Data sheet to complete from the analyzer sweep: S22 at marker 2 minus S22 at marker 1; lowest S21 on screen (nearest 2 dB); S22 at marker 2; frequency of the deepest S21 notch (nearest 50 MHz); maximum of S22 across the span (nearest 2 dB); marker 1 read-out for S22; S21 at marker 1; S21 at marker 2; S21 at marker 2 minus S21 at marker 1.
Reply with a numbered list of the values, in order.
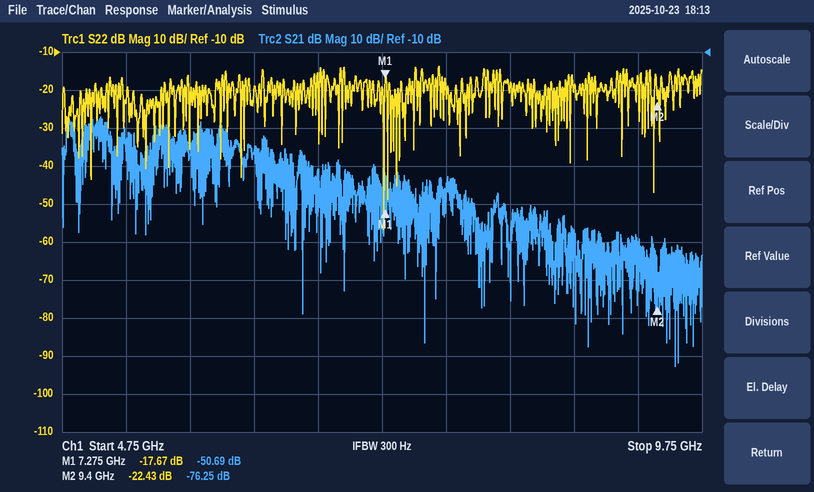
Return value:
1. -4.76 dB
2. -92 dB
3. -22.43 dB
4. 9.55 GHz
5. -14 dB
6. -17.67 dB
7. -50.69 dB
8. -76.25 dB
9. -25.56 dB
